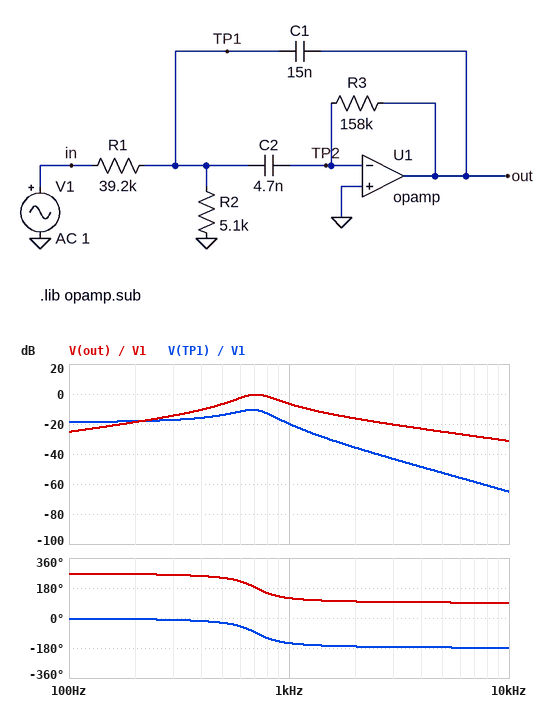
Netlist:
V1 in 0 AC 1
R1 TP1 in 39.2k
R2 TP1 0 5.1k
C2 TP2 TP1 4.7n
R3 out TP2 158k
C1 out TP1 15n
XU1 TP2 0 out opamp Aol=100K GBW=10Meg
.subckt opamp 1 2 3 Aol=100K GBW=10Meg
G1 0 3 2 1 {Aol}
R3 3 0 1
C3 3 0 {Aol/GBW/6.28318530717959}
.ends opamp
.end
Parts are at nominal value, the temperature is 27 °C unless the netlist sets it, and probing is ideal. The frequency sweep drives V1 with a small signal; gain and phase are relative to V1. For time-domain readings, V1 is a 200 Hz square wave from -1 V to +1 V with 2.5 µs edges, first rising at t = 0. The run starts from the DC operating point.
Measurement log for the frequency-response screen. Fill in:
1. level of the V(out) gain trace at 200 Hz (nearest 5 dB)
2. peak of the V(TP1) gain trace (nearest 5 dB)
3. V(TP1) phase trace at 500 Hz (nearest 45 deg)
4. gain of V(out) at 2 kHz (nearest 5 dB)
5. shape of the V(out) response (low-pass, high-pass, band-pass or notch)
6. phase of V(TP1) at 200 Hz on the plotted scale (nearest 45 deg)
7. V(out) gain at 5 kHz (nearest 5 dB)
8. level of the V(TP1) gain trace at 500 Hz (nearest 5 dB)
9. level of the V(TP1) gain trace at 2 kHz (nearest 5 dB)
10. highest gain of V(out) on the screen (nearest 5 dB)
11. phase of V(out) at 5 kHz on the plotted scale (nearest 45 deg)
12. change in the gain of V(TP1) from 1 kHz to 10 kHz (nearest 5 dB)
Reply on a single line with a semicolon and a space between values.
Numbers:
-20 dB; -10 dB; -45 deg; -15 dB; band-pass; 0 deg; -25 dB; -15 dB; -35 dB; 0 dB; 90 deg; -45 dB
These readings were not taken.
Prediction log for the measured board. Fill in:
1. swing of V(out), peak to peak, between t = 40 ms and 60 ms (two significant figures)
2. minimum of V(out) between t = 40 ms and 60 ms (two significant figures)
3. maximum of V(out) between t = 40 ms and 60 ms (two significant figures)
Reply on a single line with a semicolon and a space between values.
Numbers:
1.2 V; -590 mV; 590 mV
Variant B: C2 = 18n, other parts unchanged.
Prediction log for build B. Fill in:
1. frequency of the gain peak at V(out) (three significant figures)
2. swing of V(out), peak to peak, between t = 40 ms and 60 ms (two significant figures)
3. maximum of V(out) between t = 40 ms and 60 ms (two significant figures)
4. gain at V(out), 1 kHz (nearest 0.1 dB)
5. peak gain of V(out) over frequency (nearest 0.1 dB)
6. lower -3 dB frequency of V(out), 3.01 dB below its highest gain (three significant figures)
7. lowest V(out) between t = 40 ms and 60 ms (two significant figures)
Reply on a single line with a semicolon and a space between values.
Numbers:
363 Hz; 1.8 V; 920 mV; -10.2 dB; 6.8 dB; 306 Hz; -920 mV
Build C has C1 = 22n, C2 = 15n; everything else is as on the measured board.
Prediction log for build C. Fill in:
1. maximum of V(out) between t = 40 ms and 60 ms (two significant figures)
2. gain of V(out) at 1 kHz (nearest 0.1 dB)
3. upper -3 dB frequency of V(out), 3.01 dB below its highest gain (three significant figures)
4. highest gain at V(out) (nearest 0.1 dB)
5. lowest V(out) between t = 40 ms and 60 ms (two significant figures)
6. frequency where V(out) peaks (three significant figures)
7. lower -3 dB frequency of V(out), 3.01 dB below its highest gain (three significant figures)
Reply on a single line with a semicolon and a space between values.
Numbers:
770 mV; -13.8 dB; 389 Hz; 4.3 dB; -770 mV; 328 Hz; 276 Hz
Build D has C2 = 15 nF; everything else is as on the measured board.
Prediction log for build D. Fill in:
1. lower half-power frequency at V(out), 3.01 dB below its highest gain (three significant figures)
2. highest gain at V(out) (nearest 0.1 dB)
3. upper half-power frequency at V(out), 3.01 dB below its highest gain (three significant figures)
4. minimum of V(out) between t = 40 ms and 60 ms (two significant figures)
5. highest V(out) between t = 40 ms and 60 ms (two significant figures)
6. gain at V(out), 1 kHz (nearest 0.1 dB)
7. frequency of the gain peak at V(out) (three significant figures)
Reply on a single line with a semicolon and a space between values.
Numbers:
336 Hz; 6.1 dB; 470 Hz; -800 mV; 800 mV; -10.0 dB; 397 Hz
